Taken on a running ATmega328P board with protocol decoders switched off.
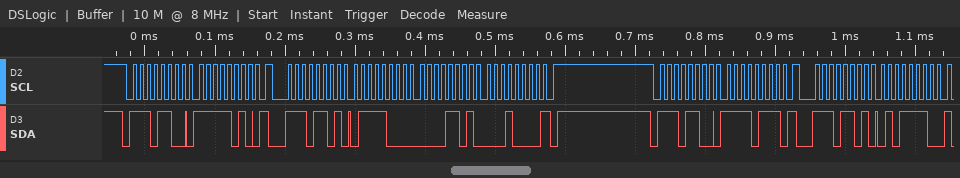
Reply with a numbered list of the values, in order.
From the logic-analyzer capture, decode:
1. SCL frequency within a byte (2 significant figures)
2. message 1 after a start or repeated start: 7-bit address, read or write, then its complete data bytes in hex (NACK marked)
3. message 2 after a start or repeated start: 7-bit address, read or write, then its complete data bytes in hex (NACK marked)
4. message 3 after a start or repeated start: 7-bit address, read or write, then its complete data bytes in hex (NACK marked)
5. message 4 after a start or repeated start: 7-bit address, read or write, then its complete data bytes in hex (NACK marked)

1. 100 kHz
2. 0x76 write: FA
3. 0x76 read: 78 0D 10 NACK
4. 0x76 write: F7
5. 0x76 read: 5E
